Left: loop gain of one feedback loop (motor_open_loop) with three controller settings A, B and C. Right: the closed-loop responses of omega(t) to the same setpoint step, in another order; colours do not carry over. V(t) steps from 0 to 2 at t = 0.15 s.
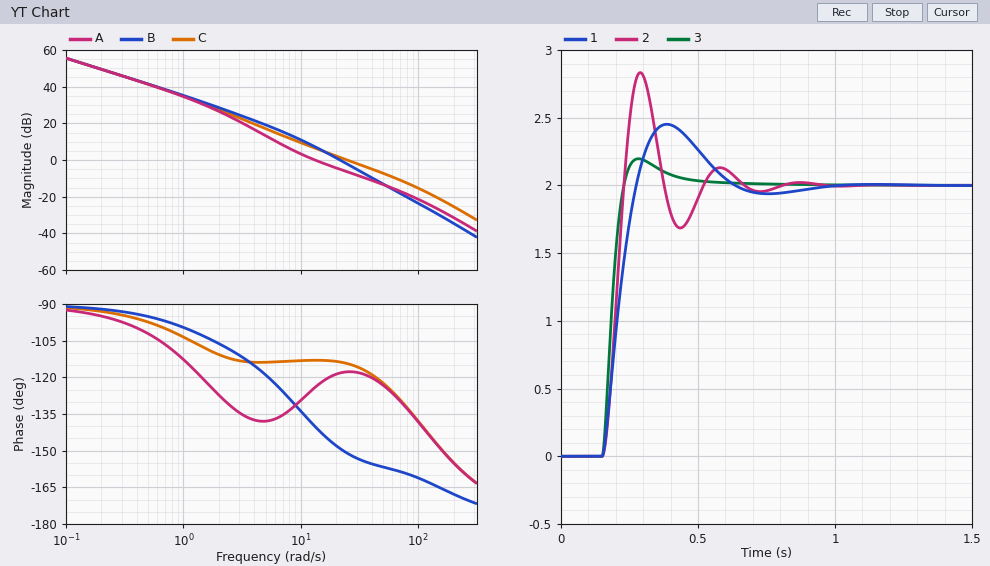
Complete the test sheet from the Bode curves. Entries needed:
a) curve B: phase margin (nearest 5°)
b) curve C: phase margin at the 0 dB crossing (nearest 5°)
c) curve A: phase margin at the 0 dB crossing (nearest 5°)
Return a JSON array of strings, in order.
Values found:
["30°", "65°", "55°"]
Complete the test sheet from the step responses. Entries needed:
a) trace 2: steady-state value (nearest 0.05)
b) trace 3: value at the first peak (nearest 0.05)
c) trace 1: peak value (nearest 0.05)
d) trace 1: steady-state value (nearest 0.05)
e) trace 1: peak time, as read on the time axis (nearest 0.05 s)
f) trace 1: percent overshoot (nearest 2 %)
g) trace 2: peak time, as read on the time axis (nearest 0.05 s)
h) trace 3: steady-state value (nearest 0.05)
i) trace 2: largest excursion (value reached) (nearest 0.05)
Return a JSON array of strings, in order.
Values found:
["2.00", "2.20", "2.45", "2.00", "0.40 s", "22 %", "0.30 s", "2.00", "2.85"]
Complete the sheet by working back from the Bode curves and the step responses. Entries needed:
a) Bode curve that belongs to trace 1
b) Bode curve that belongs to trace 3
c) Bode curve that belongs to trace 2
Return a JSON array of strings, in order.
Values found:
["A", "C", "B"]
